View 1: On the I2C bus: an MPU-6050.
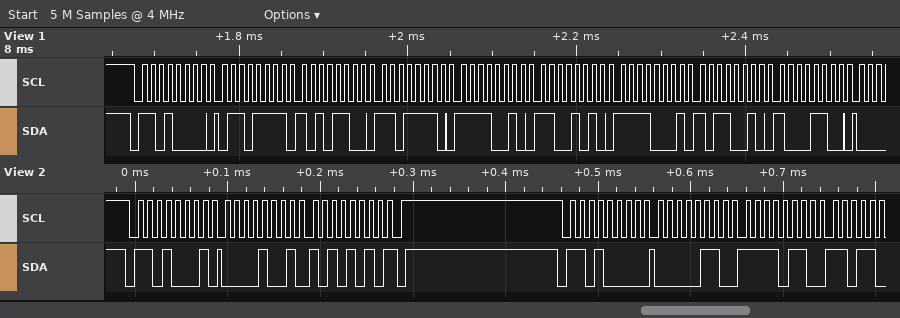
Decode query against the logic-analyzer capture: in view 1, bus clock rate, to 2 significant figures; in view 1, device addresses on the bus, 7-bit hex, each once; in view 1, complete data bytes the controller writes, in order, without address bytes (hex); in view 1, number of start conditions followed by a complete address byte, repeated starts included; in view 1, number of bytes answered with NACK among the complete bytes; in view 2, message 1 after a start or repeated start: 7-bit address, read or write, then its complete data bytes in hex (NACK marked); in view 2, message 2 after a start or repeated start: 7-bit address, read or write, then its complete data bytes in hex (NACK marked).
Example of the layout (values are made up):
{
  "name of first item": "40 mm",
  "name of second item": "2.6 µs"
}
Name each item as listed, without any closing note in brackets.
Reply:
{
  "in view 1, bus clock rate, to 2 significant figures": "100 kHz",
  "in view 1, device addresses on the bus, 7-bit hex, each once": "0x68",
  "in view 1, complete data bytes the controller writes, in order, without address bytes": "6F AC DE F2 CA F1 B2 8C",
  "in view 1, number of start conditions followed by a complete address byte, repeated starts included": "1",
  "in view 1, number of bytes answered with NACK among the complete bytes": "0",
  "in view 2, message 1 after a start or repeated start: 7-bit address, read or write, then its complete data bytes in hex": "0x68 read: 09 AA NACK",
  "in view 2, message 2 after a start or repeated start: 7-bit address, read or write, then its complete data bytes in hex": "0x68 write: 06 F6"
}
